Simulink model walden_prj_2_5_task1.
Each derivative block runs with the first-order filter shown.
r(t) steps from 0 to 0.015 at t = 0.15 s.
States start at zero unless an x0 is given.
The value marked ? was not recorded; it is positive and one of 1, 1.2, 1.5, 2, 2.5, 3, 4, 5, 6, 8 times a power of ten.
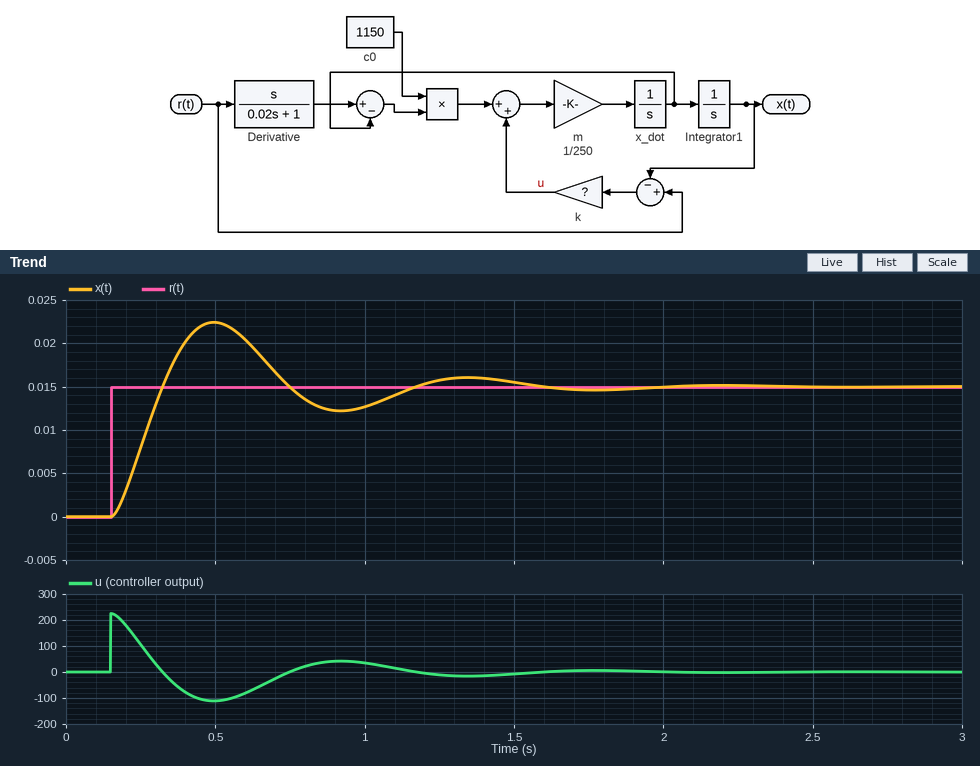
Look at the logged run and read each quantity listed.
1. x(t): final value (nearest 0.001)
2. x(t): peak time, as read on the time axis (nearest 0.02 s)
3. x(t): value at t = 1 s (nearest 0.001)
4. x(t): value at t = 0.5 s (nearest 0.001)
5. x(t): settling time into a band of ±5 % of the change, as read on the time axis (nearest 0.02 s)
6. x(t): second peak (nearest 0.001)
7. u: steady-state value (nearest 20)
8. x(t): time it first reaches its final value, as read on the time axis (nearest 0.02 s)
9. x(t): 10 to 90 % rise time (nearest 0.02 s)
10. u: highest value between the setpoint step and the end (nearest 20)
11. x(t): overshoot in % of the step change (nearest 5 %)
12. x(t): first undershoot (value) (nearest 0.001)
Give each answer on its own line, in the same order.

0.015
0.50 s
0.013
0.022
1.46 s
0.016
0
0.32 s
0.12 s
220
50 %
0.012
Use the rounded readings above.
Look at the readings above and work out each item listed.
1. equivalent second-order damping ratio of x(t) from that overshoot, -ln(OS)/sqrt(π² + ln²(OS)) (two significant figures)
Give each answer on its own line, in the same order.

0.22
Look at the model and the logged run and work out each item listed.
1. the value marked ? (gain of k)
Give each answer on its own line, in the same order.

15000
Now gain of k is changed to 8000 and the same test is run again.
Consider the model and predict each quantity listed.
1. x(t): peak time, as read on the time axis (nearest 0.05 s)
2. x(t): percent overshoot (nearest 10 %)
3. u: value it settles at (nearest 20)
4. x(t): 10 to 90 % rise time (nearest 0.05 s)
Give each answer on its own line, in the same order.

0.60 s
40 %
0
0.15 s
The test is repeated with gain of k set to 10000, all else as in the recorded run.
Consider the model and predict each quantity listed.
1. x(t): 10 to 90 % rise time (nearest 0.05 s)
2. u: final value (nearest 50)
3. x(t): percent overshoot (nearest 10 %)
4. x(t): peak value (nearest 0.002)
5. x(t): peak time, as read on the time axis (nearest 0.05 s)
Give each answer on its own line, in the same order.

0.15 s
0
40 %
0.022
0.55 s
